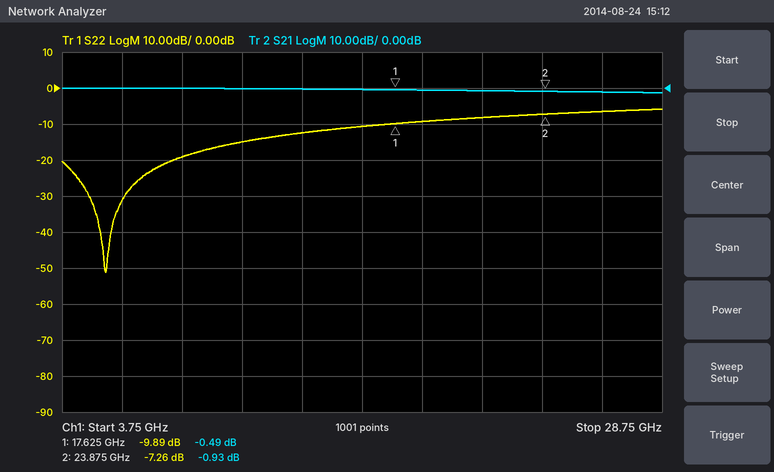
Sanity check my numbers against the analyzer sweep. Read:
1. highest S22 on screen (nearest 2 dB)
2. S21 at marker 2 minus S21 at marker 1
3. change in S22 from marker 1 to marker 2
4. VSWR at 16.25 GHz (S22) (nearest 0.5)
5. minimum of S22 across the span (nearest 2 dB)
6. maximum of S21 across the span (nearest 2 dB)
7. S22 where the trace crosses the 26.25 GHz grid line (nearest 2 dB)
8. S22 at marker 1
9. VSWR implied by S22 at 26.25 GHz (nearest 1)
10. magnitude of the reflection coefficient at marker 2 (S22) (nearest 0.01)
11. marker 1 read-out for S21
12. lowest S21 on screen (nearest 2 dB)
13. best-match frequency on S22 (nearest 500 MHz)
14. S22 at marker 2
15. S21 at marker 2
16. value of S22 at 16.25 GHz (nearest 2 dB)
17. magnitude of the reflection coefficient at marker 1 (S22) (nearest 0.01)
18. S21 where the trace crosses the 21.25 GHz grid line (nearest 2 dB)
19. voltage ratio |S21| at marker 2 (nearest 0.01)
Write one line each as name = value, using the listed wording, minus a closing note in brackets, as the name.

highest S22 on screen = -6 dB
S21 at marker 2 minus S21 at marker 1 = -0.44 dB
change in S22 from marker 1 to marker 2 = 2.63 dB
VSWR at 16.25 GHz (S22) = 2.0
minimum of S22 across the span = -52 dB
maximum of S21 across the span = 0 dB
S22 where the trace crosses the 26.25 GHz grid line = -6 dB
S22 at marker 1 = -9.89 dB
VSWR implied by S22 at 26.25 GHz = 3
magnitude of the reflection coefficient at marker 2 (S22) = 0.43
marker 1 read-out for S21 = -0.49 dB
lowest S21 on screen = -2 dB
best-match frequency on S22 = 5.5 GHz
S22 at marker 2 = -7.26 dB
S21 at marker 2 = -0.93 dB
value of S22 at 16.25 GHz = -10 dB
magnitude of the reflection coefficient at marker 1 (S22) = 0.32
S21 where the trace crosses the 21.25 GHz grid line = 0 dB
voltage ratio |S21| at marker 2 = 0.90
